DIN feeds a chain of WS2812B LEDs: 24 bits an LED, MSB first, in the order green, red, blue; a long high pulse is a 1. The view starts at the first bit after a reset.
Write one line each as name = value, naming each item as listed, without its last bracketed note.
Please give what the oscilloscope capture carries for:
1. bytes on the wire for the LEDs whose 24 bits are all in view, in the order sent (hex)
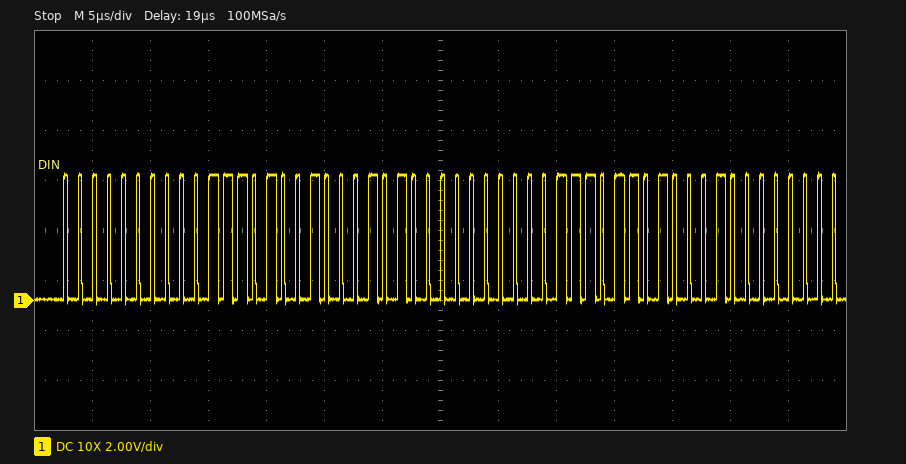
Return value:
bytes on the wire for the LEDs whose 24 bits are all in view, in the order sent = 00 3A 45 00 3B 44
